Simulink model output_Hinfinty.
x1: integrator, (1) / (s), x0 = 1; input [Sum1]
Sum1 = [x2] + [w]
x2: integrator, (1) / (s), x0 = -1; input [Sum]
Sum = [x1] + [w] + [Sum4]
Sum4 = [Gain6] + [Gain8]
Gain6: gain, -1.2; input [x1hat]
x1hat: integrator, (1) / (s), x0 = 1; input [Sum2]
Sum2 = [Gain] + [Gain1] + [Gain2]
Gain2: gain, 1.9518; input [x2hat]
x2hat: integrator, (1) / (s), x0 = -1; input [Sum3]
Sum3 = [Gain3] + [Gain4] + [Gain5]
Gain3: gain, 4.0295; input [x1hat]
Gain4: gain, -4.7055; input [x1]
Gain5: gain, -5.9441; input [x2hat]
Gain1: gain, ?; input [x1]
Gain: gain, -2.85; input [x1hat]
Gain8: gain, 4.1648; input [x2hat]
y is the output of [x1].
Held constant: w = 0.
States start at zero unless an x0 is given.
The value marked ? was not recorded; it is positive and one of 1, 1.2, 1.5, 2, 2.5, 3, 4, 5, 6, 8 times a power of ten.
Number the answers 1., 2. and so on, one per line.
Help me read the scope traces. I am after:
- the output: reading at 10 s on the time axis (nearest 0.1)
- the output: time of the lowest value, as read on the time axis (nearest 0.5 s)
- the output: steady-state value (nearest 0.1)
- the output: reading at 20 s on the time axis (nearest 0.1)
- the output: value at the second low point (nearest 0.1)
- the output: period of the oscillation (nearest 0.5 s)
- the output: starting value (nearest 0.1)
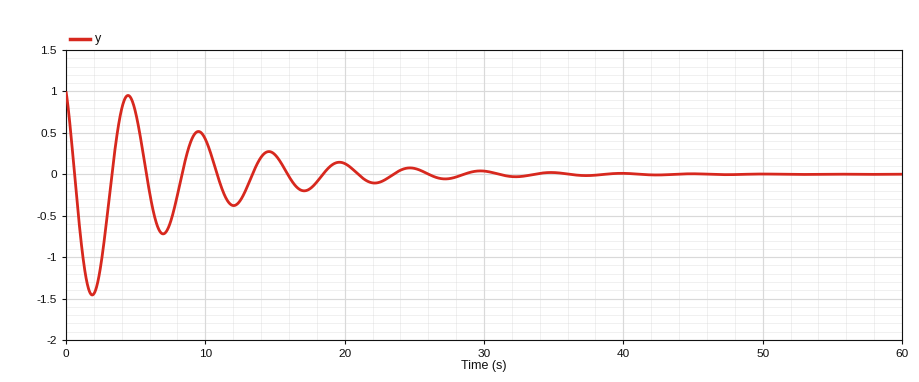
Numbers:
1. 0.4
2. 2.0 s
3. 0.0
4. 0.1
5. -0.7
6. 5.0 s
7. 1.0
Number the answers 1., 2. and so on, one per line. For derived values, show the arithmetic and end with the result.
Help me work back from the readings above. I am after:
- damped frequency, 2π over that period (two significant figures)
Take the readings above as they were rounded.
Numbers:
1. 2π / 5 = 1.3 rad/s
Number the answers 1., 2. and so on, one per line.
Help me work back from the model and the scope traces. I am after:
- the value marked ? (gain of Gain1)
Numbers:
1. 3
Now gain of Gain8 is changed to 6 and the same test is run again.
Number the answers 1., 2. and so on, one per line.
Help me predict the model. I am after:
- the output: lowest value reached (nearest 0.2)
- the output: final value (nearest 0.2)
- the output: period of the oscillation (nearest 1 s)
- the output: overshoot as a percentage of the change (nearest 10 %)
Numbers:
1. -1.2
2. 0.0
3. 4 s
4. 130 %
